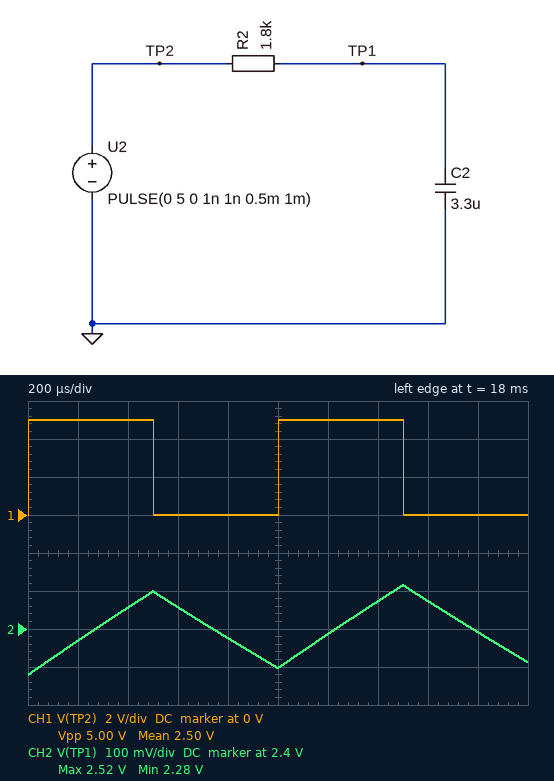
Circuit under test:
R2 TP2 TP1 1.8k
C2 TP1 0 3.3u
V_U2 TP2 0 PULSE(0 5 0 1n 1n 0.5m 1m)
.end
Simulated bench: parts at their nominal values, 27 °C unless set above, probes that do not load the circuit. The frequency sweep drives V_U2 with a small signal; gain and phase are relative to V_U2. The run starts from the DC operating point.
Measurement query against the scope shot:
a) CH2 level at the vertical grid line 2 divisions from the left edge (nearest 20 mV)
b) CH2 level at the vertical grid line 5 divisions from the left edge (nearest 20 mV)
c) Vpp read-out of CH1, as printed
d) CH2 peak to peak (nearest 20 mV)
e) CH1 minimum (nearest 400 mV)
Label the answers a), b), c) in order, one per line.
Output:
a) 2.46 V
b) 2.30 V
c) 5.00 V
d) 240 mV
e) 0 V
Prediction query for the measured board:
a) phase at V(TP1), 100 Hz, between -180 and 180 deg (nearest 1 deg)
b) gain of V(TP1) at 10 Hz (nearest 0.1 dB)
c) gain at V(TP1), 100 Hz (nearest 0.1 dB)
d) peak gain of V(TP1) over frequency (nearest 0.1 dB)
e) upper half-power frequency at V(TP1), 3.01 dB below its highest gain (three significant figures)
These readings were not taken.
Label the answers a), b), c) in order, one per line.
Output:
a) -75 deg
b) -0.6 dB
c) -11.7 dB
d) 0 dB
e) 26.8 Hz
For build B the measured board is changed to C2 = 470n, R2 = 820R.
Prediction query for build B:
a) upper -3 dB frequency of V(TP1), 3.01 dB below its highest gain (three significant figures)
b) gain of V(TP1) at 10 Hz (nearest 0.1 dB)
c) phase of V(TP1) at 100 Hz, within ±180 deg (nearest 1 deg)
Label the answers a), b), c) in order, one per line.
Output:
a) 413 Hz
b) 0 dB
c) -14 deg
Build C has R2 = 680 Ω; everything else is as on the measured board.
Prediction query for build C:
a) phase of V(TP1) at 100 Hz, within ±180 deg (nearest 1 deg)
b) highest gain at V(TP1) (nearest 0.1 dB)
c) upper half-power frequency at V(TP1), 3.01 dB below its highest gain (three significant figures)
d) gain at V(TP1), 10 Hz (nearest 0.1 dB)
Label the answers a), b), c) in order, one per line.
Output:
a) -55 deg
b) 0 dB
c) 70.9 Hz
d) -0.1 dB
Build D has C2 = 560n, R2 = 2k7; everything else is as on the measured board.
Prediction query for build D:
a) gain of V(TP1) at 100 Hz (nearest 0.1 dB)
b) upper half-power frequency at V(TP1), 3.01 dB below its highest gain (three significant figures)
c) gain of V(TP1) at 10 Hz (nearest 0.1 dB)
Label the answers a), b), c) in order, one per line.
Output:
a) -2.8 dB
b) 105 Hz
c) 0 dB
